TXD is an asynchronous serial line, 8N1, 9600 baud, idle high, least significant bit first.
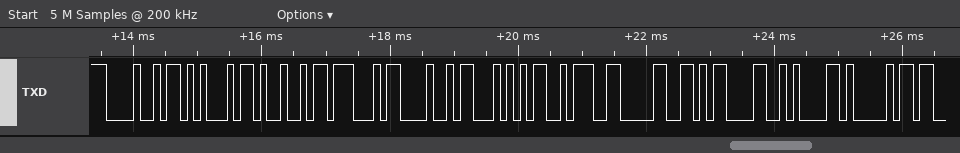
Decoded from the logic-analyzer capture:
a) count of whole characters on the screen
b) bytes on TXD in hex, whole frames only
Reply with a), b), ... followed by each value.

a) 11
b) 0x48 0x45 0x49 0x47 0x48 0x54 0x3A 0x30 0x0D 0x0A 0x41
